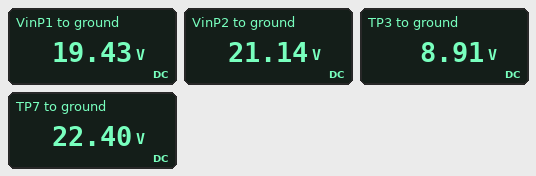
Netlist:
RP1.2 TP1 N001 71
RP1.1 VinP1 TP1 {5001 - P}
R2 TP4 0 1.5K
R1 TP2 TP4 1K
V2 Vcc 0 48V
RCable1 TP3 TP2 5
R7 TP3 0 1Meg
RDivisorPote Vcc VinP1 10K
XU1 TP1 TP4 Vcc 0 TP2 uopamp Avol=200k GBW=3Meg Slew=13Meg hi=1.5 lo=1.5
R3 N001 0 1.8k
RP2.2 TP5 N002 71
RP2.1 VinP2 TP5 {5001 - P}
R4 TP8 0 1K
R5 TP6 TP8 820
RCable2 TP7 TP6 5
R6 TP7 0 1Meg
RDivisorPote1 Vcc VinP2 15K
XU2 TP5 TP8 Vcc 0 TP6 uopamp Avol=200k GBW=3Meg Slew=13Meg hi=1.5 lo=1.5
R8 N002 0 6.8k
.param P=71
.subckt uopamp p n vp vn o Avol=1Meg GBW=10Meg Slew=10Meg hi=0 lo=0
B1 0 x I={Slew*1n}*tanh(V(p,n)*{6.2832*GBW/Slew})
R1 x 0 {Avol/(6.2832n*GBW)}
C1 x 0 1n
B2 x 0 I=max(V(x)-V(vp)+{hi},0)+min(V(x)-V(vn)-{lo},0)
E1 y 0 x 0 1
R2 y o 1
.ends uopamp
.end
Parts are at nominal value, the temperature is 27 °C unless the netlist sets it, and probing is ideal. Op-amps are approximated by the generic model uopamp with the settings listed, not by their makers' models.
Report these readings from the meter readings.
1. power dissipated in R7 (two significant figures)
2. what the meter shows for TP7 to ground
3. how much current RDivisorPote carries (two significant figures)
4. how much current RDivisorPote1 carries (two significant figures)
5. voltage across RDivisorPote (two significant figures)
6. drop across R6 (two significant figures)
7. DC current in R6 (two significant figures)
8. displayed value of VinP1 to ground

79 µW
22.40 V
2.9 mA
1.8 mA
29 V
22 V
22 µA
19.43 V
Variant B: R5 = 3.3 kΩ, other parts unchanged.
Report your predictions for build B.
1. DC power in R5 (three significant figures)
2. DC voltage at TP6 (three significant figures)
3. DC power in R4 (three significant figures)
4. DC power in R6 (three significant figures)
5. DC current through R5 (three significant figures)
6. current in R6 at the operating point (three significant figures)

386 mW
46.5 V
117 mW
2.16 mW
10.8 mA
46.5 µA
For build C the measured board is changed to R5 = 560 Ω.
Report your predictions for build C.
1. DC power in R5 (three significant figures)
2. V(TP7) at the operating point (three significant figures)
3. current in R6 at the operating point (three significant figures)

84.8 mW
19.2 V
19.2 µA
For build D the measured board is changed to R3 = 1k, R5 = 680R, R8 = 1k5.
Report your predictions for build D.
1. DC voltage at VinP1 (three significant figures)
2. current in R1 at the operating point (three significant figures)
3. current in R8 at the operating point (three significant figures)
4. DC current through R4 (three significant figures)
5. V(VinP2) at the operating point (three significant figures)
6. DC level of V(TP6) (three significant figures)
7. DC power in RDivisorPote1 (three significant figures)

18.0 V
2.14 mA
2.23 mA
3.51 mA
14.5 V
5.89 V
74.8 mW
